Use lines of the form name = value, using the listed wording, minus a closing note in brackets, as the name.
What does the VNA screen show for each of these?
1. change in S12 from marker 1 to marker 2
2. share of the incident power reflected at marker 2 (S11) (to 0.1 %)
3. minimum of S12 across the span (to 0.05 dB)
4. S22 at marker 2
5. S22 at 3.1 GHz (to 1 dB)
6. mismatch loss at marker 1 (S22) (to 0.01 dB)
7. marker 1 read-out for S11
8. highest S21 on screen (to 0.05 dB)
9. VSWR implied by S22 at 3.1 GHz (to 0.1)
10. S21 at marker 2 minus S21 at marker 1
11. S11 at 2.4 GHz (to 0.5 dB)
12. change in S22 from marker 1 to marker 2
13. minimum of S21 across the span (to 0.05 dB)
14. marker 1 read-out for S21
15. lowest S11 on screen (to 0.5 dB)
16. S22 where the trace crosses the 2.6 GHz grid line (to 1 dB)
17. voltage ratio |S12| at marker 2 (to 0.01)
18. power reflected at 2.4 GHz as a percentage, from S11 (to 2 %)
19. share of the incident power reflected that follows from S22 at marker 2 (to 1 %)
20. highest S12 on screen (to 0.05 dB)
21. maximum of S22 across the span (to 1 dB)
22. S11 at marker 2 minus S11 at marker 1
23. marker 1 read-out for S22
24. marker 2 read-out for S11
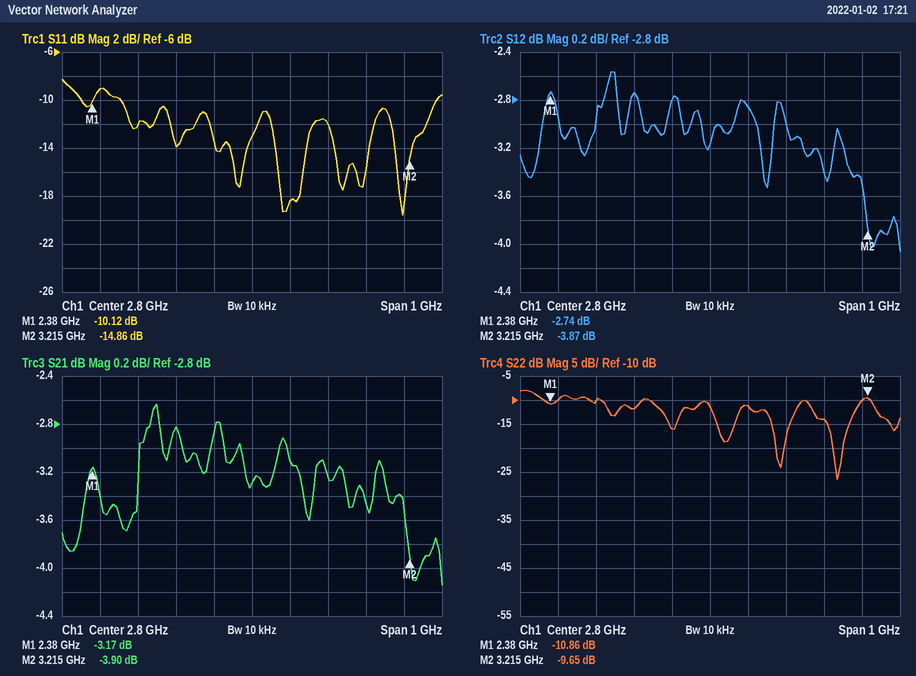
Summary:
change in S12 from marker 1 to marker 2 = -1.13 dB
share of the incident power reflected at marker 2 (S11) = 3.3 %
minimum of S12 across the span = -4.05 dB
S22 at marker 2 = -9.65 dB
S22 at 3.1 GHz = -14 dB
mismatch loss at marker 1 (S22) = 0.37 dB
marker 1 read-out for S11 = -10.12 dB
highest S21 on screen = -2.65 dB
VSWR implied by S22 at 3.1 GHz = 1.5
S21 at marker 2 minus S21 at marker 1 = -0.73 dB
S11 at 2.4 GHz = -9.0 dB
change in S22 from marker 1 to marker 2 = 1.21 dB
minimum of S21 across the span = -4.15 dB
marker 1 read-out for S21 = -3.17 dB
lowest S11 on screen = -19.5 dB
S22 where the trace crosses the 2.6 GHz grid line = -12 dB
voltage ratio |S12| at marker 2 = 0.64
power reflected at 2.4 GHz as a percentage, from S11 = 12 %
share of the incident power reflected that follows from S22 at marker 2 = 11 %
highest S12 on screen = -2.55 dB
maximum of S22 across the span = -8 dB
S11 at marker 2 minus S11 at marker 1 = -4.74 dB
marker 1 read-out for S22 = -10.86 dB
marker 2 read-out for S11 = -14.86 dB
